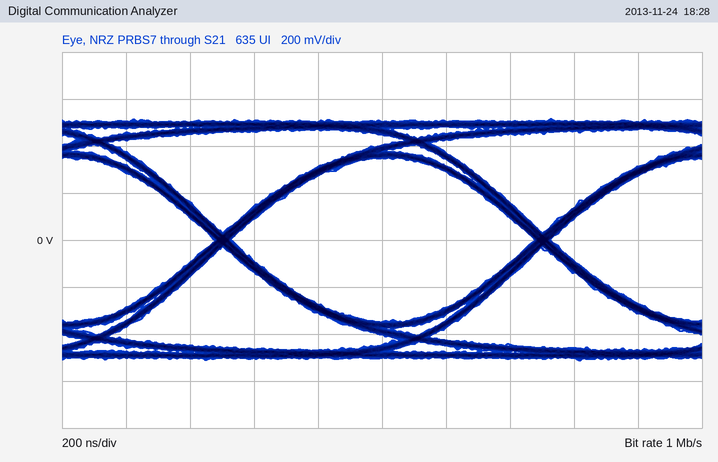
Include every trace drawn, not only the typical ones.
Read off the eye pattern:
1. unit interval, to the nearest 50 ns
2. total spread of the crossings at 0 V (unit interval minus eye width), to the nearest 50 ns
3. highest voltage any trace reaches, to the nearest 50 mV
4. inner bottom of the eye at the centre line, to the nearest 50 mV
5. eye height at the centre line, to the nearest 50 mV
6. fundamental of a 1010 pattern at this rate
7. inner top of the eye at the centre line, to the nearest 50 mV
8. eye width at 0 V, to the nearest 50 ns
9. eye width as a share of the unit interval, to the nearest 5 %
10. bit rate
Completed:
1.00 µs
50 ns
500 mV
-350 mV
700 mV
500 kHz
350 mV
950 ns
95 %
1 Mb/s
